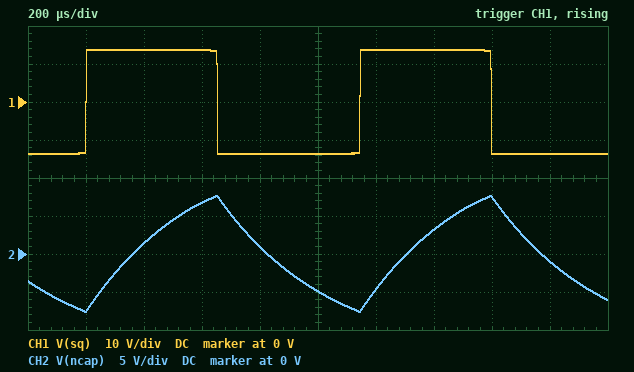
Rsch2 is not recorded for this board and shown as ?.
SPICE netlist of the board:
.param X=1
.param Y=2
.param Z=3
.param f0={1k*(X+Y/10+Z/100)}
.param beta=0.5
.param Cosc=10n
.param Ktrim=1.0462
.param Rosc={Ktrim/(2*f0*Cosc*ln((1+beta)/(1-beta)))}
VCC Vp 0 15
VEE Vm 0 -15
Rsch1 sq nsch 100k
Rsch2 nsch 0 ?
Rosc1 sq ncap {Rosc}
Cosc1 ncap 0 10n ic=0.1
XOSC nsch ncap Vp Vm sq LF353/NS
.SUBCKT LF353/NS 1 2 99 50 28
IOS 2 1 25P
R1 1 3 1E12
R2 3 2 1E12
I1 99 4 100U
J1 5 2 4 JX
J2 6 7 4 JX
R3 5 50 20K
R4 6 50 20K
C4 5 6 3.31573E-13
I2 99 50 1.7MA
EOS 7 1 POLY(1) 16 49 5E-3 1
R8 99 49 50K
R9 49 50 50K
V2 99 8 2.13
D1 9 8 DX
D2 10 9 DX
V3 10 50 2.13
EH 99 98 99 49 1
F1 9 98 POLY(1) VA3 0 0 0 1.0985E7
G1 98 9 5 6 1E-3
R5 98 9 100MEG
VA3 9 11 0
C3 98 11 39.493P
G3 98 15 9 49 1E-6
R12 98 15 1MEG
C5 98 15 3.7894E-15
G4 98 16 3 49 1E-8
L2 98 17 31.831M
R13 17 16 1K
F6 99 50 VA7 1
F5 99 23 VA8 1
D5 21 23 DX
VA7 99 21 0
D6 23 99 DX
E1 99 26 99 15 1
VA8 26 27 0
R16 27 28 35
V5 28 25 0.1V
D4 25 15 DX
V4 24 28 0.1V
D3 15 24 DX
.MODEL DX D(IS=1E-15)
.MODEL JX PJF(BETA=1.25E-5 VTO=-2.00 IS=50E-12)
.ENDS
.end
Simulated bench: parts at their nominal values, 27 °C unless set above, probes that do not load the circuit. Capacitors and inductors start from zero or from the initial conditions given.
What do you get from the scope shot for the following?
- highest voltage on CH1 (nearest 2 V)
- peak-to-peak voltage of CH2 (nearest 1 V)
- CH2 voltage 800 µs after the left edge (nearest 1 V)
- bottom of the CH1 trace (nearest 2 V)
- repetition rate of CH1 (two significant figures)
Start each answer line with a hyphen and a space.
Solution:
- 14 V
- 15 V
- 1 V
- -14 V
- 1.1 kHz
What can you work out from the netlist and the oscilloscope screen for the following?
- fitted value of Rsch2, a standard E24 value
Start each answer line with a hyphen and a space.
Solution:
- 130 kΩ
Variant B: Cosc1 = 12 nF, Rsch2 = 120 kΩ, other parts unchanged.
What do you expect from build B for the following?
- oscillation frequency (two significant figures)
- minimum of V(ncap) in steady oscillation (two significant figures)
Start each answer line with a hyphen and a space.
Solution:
- 920 Hz
- -7.3 V
